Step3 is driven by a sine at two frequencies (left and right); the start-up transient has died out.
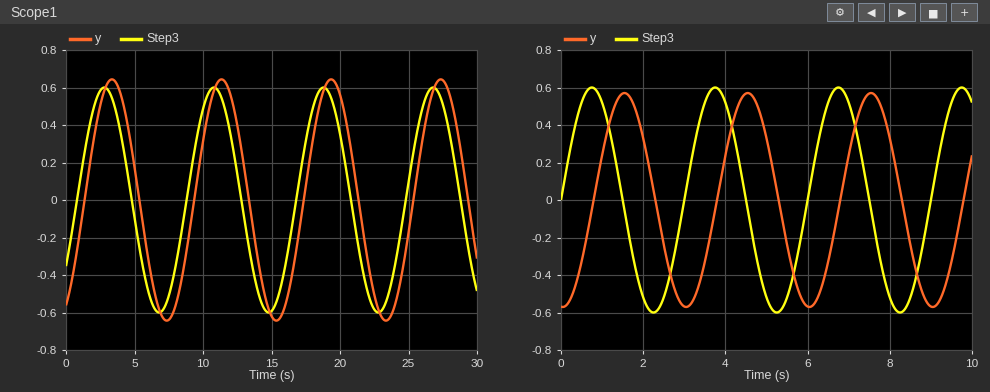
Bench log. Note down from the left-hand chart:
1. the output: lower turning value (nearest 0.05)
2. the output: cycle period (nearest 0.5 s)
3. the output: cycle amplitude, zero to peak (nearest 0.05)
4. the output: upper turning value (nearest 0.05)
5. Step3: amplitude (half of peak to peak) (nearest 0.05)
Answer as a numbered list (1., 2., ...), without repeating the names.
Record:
1. -0.65
2. 8.0 s
3. 0.65
4. 0.65
5. 0.60
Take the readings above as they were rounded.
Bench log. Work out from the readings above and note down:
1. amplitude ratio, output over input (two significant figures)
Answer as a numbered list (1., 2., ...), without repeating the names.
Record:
1. 1.1
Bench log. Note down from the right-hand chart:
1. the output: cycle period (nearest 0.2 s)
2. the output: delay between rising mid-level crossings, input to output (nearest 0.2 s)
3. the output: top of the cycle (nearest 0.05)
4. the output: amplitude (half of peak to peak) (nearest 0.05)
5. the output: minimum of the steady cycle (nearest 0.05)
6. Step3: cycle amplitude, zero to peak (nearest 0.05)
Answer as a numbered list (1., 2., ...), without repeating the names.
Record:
1. 3.0 s
2. 0.8 s
3. 0.55
4. 0.55
5. -0.55
6. 0.60
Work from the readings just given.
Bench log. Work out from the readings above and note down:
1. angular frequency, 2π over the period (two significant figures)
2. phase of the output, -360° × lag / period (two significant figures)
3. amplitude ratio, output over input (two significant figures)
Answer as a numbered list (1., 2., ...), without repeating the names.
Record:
1. 2.1 rad/s
2. -96°
3. 0.92
